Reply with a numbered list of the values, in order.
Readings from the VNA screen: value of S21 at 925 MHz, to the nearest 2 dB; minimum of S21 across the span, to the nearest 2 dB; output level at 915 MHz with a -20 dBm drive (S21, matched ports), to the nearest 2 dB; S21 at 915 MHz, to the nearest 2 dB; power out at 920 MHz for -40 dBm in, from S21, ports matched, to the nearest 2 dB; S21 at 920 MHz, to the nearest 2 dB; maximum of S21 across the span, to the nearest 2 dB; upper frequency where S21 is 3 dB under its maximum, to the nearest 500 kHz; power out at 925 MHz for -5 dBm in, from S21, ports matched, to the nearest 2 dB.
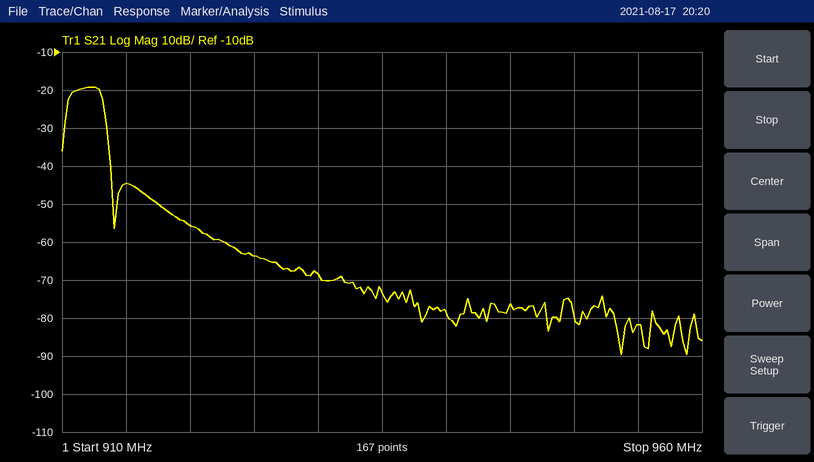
1. -64 dB
2. -90 dB
3. -64 dBm
4. -44 dB
5. -96 dBm
6. -56 dB
7. -20 dB
8. 913.0 MHz
9. -68 dBm
